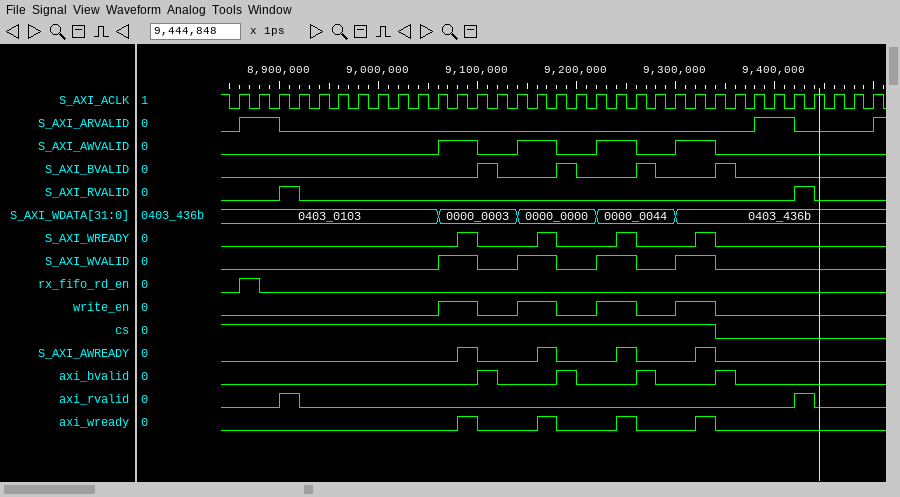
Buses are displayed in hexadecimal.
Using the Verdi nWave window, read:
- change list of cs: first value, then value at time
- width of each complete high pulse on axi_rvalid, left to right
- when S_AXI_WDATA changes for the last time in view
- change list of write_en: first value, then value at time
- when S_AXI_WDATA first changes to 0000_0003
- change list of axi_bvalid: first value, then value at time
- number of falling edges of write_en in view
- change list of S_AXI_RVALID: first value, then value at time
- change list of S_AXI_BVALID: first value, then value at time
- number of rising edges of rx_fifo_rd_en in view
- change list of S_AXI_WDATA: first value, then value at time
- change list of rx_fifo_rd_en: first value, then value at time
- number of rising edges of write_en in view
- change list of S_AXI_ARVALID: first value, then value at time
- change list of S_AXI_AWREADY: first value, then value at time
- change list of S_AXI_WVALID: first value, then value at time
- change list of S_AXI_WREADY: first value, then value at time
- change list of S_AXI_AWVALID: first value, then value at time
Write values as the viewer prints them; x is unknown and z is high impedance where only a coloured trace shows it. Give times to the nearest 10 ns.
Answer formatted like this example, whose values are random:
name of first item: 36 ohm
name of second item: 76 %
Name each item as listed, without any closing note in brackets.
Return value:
change list of cs: first value, then value at time: 1, 0 at 9340 ns
width of each complete high pulse on axi_rvalid, left to right: 20 ns, 20 ns
when S_AXI_WDATA changes for the last time in view: 9300 ns
change list of write_en: first value, then value at time: 0, 1 at 9060 ns, 0 at 9100 ns, 1 at 9140 ns, 0 at 9180 ns, 1 at 9220 ns, 0 at 9260 ns, 1 at 9300 ns, 0 at 9340 ns
when S_AXI_WDATA first changes to 0000_0003: 9060 ns
change list of axi_bvalid: first value, then value at time: 0, 1 at 9100 ns, 0 at 9120 ns, 1 at 9180 ns, 0 at 9200 ns, 1 at 9260 ns, 0 at 9280 ns, 1 at 9340 ns, 0 at 9360 ns
number of falling edges of write_en in view: 4
change list of S_AXI_RVALID: first value, then value at time: 0, 1 at 8900 ns, 0 at 8920 ns, 1 at 9420 ns, 0 at 9440 ns
change list of S_AXI_BVALID: first value, then value at time: 0, 1 at 9100 ns, 0 at 9120 ns, 1 at 9180 ns, 0 at 9200 ns, 1 at 9260 ns, 0 at 9280 ns, 1 at 9340 ns, 0 at 9360 ns
number of rising edges of rx_fifo_rd_en in view: 1
change list of S_AXI_WDATA: first value, then value at time: 0403_0103, 0000_0003 at 9060 ns, 0000_0000 at 9140 ns, 0000_0044 at 9220 ns, 0403_436b at 9300 ns
change list of rx_fifo_rd_en: first value, then value at time: 0, 1 at 8860 ns, 0 at 8880 ns
number of rising edges of write_en in view: 4
change list of S_AXI_ARVALID: first value, then value at time: 0, 1 at 8860 ns, 0 at 8900 ns, 1 at 9380 ns, 0 at 9420 ns, 1 at 9500 ns
change list of S_AXI_AWREADY: first value, then value at time: 0, 1 at 9080 ns, 0 at 9100 ns, 1 at 9160 ns, 0 at 9180 ns, 1 at 9240 ns, 0 at 9260 ns, 1 at 9320 ns, 0 at 9340 ns
change list of S_AXI_WVALID: first value, then value at time: 0, 1 at 9060 ns, 0 at 9100 ns, 1 at 9140 ns, 0 at 9180 ns, 1 at 9220 ns, 0 at 9260 ns, 1 at 9300 ns, 0 at 9340 ns
change list of S_AXI_WREADY: first value, then value at time: 0, 1 at 9080 ns, 0 at 9100 ns, 1 at 9160 ns, 0 at 9180 ns, 1 at 9240 ns, 0 at 9260 ns, 1 at 9320 ns, 0 at 9340 ns
change list of S_AXI_AWVALID: first value, then value at time: 0, 1 at 9060 ns, 0 at 9100 ns, 1 at 9140 ns, 0 at 9180 ns, 1 at 9220 ns, 0 at 9260 ns, 1 at 9300 ns, 0 at 9340 ns
